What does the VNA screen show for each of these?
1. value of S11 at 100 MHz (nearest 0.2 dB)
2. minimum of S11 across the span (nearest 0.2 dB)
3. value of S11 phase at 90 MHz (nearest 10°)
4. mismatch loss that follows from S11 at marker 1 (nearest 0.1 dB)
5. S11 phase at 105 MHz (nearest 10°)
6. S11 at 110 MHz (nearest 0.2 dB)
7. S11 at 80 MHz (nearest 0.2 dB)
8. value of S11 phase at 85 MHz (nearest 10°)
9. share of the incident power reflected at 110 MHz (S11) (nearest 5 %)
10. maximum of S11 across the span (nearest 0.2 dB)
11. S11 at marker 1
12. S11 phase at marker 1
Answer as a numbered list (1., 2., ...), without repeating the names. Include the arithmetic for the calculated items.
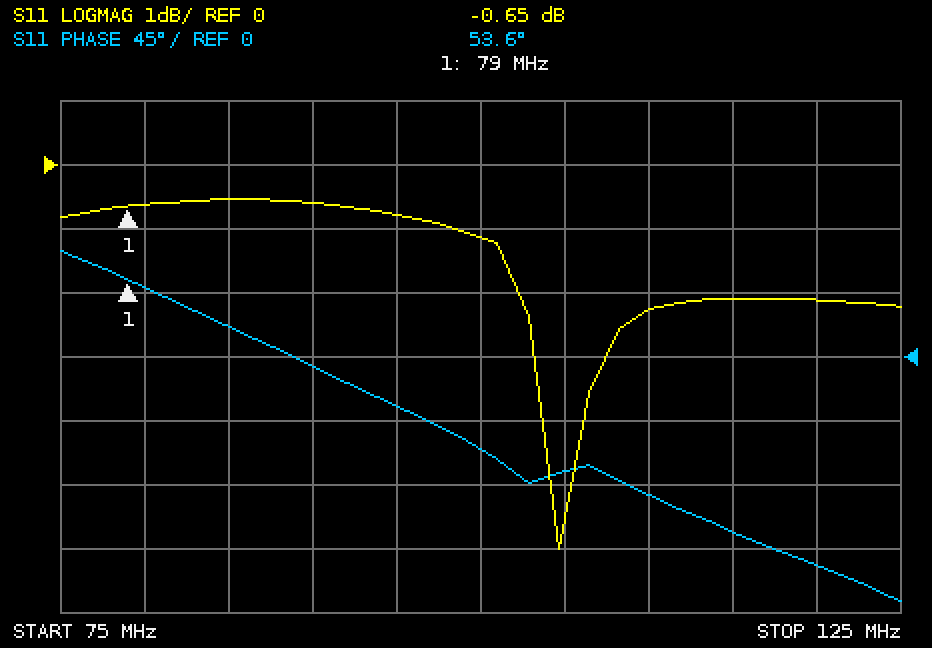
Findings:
1. -1.2 dB
2. -6.0 dB
3. -10°
4. −10 log10(1 − 10^(-0.65/10)) ≈ 8.6 dB
5. -80°
6. -2.2 dB
7. -0.6 dB
8. 20°
9. 10^(-2.2/10) ≈ 60 %
10. -0.6 dB
11. -0.65 dB
12. 53.6°
